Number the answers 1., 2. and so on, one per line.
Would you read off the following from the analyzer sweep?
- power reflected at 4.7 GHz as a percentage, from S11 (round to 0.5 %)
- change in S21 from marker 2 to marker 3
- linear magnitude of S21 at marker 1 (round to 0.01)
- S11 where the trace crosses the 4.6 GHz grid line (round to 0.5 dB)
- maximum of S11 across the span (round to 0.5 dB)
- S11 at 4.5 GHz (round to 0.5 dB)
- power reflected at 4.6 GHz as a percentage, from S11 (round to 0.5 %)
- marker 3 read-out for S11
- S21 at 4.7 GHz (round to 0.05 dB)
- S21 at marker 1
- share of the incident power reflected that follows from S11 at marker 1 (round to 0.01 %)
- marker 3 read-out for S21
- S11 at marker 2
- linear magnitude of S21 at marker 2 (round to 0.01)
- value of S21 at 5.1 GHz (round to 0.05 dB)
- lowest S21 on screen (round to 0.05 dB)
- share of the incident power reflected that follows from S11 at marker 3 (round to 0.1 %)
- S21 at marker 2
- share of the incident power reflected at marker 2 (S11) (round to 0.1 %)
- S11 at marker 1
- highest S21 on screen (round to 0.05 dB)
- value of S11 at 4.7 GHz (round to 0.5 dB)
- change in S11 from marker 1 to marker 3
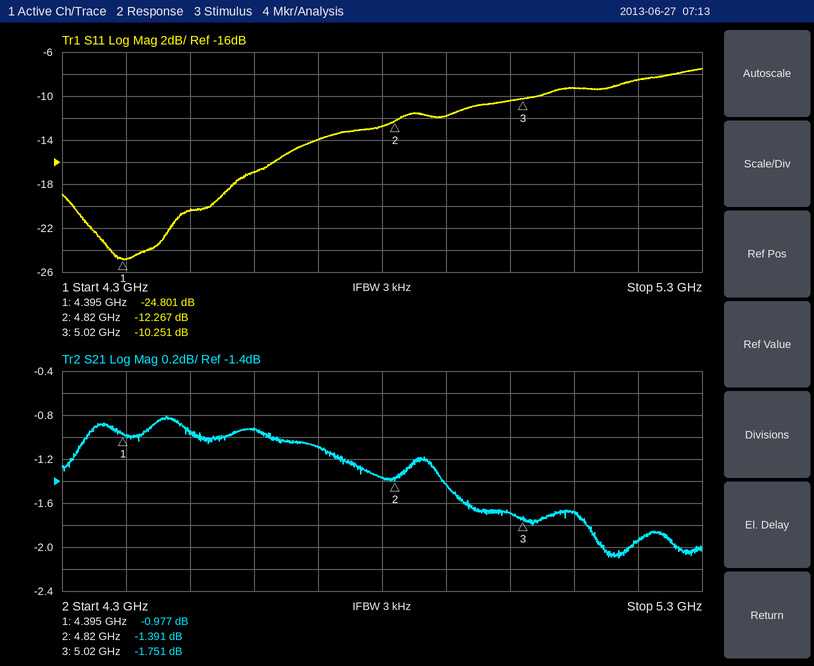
1. 4.0 %
2. -0.360 dB
3. 0.89
4. -17.0 dB
5. -7.5 dB
6. -20.5 dB
7. 2.0 %
8. -10.251 dB
9. -1.10 dB
10. -0.977 dB
11. 0.33 %
12. -1.751 dB
13. -12.267 dB
14. 0.85
15. -1.70 dB
16. -2.10 dB
17. 9.4 %
18. -1.391 dB
19. 5.9 %
20. -24.801 dB
21. -0.80 dB
22. -14.0 dB
23. 14.550 dB
